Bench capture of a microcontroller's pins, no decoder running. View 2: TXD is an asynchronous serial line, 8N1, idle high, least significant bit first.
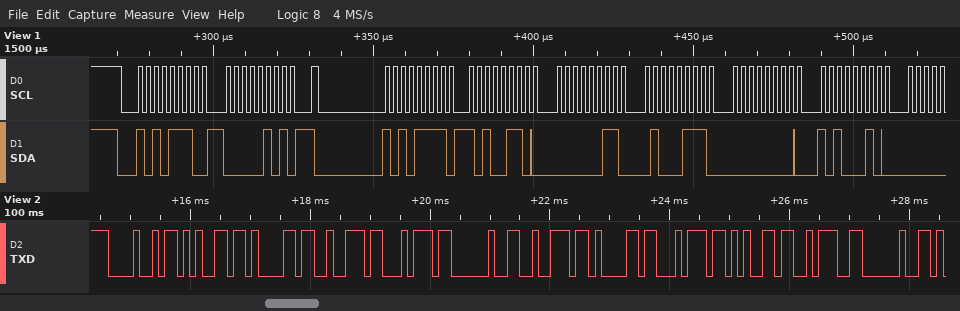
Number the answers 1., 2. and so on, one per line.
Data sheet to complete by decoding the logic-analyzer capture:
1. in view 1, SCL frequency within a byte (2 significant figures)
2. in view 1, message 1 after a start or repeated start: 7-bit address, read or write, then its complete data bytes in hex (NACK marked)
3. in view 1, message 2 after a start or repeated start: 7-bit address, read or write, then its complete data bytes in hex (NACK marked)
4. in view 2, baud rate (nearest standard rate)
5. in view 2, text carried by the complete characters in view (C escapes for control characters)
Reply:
1. 400 kHz
2. 0x57 write: 05
3. 0x57 read: A6 03 47 00 A2
4. 9600 baud
5. "Heart rate: "
